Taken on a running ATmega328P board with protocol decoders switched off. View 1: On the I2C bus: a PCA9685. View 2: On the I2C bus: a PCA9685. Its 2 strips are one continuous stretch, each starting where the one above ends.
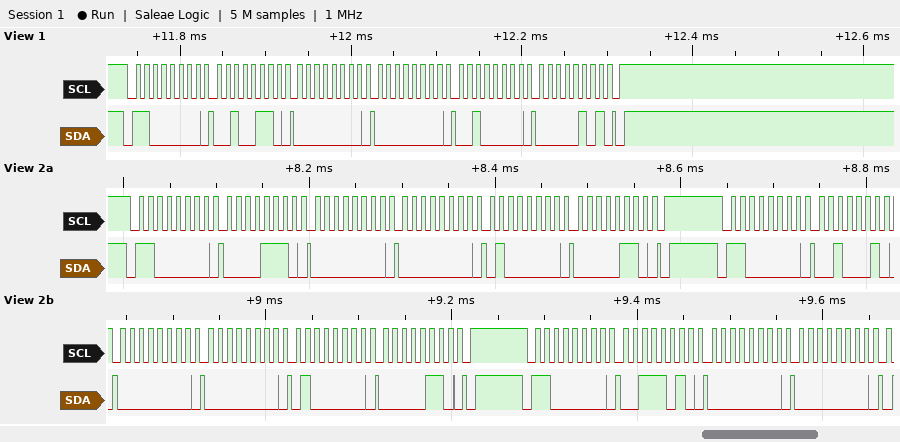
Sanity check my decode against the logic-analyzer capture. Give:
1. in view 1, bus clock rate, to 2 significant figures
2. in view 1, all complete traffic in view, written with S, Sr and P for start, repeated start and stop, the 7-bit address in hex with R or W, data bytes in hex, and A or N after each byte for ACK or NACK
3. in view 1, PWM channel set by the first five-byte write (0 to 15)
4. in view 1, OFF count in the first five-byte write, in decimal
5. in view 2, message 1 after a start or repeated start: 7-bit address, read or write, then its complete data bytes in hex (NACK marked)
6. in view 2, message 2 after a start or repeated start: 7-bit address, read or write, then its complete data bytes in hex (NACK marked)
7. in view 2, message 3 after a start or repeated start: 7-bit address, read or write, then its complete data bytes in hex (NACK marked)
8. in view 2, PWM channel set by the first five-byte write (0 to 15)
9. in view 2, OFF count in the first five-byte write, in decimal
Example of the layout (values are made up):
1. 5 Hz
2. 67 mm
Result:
1. 100 kHz
2. S 60W A 26 A 00 A 00 A 20 A 05 A P
3. 8
4. 1312
5. 0x60 write: 0E 00 00 40 06
6. 0x60 write: 22 00 00 40 06
7. 0x60 write: 3A 00 00
8. 2
9. 1600
